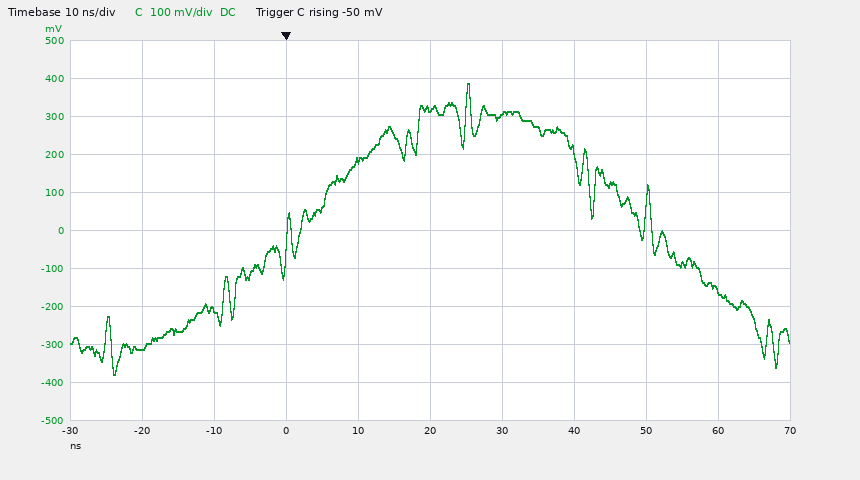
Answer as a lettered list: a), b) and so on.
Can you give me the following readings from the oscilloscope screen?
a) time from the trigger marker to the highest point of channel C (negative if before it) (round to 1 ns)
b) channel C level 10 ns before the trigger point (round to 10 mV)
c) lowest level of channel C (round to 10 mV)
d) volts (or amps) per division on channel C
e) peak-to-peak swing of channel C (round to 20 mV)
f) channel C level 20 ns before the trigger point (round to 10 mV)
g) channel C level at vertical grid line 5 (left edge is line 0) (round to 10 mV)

a) +25 ns
b) -210 mV
c) -380 mV
d) 100 mV
e) 760 mV
f) -310 mV
g) 320 mV
